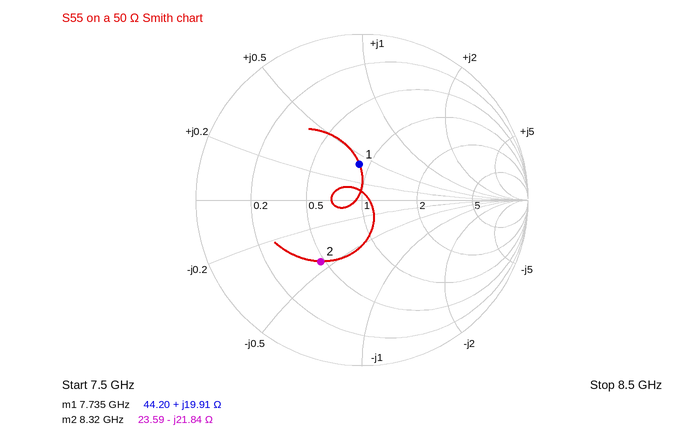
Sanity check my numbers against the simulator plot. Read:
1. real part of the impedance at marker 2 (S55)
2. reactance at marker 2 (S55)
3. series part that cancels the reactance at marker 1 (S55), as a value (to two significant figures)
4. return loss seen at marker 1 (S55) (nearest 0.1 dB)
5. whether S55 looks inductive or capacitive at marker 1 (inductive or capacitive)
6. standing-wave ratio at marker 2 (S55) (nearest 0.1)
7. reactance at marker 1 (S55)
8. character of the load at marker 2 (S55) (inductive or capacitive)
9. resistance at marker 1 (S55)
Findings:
23.59 Ω
-21.84 Ω
1.0 pF
13.3 dB
inductive
2.6
+19.91 Ω
capacitive
44.20 Ω
